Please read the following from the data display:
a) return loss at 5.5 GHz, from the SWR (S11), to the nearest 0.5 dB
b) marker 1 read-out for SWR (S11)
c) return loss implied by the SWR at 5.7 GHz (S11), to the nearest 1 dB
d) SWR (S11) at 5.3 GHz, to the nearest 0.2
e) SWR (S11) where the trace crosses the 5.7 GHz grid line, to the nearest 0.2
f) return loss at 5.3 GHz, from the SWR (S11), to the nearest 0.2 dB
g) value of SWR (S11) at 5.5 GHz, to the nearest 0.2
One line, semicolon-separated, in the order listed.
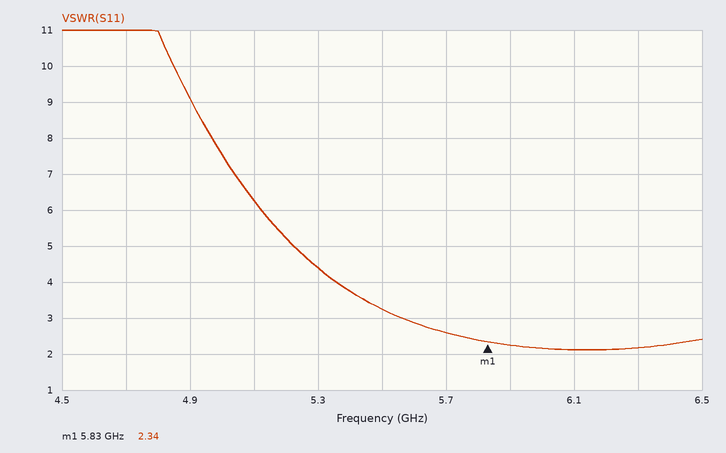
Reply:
5.5 dB; 2.34; 7 dB; 4.4; 2.6; 4.0 dB; 3.2
